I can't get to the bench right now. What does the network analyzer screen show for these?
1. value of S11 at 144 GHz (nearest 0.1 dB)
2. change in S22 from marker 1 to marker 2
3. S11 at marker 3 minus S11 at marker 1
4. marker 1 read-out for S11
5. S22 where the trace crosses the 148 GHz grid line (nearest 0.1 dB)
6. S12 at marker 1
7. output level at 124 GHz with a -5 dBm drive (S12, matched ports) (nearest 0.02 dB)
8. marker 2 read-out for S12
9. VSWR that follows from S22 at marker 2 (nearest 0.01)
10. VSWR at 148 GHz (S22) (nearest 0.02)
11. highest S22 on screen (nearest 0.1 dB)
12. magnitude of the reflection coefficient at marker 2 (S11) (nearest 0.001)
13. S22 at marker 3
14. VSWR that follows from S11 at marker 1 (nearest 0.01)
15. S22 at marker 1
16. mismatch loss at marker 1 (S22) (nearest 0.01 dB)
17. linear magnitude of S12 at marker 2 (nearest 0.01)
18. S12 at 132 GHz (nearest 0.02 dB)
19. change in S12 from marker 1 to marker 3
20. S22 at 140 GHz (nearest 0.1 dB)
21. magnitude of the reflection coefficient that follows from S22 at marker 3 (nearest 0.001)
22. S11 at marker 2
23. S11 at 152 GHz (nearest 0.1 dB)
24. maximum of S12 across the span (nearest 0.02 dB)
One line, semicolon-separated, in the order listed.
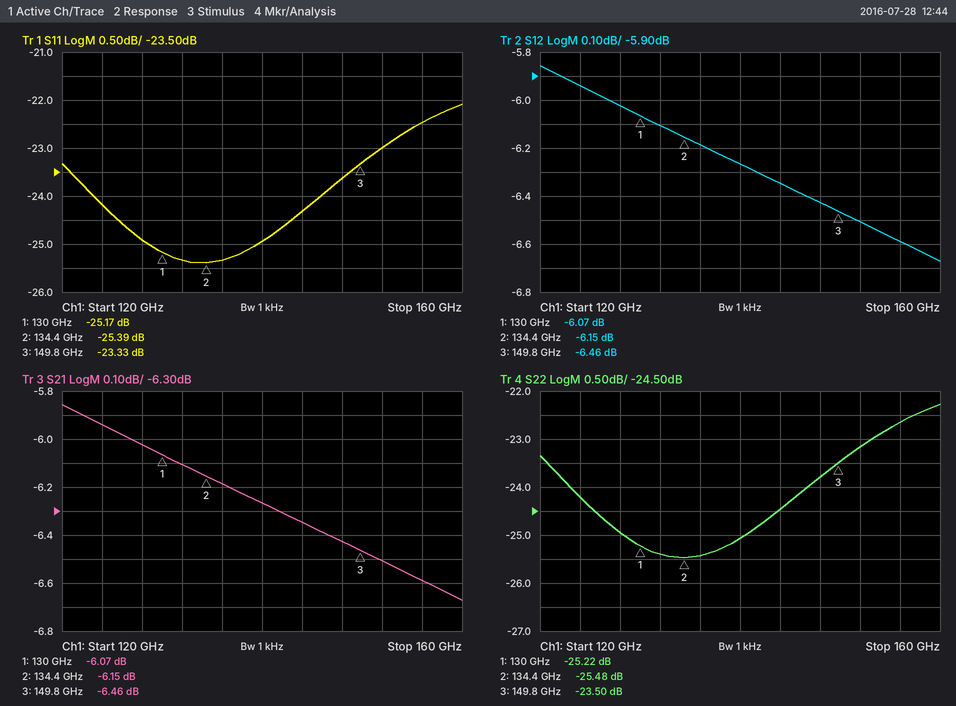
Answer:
-24.3 dB; -0.26 dB; 1.84 dB; -25.17 dB; -23.8 dB; -6.07 dB; -10.94 dBm; -6.15 dB; 1.11; 1.14; -22.3 dB; 0.054; -23.50 dB; 1.12; -25.22 dB; 0.01 dB; 0.49; -6.10 dB; -0.39 dB; -25.1 dB; 0.067; -25.39 dB; -23.0 dB; -5.86 dB
